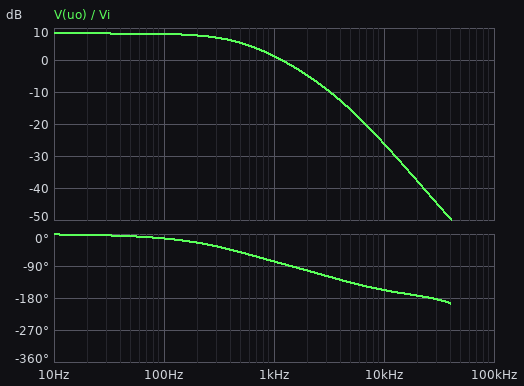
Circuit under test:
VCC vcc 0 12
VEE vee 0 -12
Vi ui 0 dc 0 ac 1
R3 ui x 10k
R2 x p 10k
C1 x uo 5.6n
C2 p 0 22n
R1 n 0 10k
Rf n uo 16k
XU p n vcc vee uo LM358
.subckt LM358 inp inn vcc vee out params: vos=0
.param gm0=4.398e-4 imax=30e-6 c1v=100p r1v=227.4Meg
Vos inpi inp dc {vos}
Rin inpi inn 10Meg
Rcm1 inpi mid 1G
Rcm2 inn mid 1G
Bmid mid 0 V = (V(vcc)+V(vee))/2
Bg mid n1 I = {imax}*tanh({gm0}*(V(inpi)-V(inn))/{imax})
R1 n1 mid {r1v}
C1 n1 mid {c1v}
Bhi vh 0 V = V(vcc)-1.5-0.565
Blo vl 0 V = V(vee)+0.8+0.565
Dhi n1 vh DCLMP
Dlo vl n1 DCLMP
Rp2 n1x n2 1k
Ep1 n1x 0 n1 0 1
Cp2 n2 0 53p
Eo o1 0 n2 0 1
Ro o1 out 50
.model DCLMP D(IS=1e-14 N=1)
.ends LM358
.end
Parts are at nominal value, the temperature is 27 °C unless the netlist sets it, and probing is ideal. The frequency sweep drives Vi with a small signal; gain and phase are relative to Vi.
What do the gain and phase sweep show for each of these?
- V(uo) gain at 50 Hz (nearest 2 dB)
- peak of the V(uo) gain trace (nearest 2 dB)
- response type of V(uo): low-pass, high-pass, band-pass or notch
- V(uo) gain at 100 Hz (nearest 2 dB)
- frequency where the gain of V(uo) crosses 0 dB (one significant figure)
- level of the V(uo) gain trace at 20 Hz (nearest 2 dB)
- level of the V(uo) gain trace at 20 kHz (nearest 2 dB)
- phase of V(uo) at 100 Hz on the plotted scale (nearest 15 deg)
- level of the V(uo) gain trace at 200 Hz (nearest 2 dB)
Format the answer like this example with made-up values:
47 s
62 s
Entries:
8 dB
8 dB
low-pass
8 dB
1 kHz
8 dB
-38 dB
-15 deg
8 dB
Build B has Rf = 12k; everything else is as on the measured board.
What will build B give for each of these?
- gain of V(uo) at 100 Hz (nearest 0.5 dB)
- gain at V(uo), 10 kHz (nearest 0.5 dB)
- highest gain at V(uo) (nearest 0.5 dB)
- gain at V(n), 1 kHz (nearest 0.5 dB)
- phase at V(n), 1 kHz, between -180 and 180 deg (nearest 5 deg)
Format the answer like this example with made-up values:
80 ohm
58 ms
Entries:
6.5 dB
-27.5 dB
7.0 dB
-7.5 dB
-80 deg
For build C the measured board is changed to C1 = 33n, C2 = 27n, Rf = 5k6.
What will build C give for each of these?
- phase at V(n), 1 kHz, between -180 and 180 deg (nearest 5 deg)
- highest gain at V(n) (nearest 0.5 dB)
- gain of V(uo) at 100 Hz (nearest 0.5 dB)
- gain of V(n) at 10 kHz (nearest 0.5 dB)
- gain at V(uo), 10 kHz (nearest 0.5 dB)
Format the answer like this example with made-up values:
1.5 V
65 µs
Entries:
-140 deg
0.5 dB
4.0 dB
-51.0 dB
-47.0 dB
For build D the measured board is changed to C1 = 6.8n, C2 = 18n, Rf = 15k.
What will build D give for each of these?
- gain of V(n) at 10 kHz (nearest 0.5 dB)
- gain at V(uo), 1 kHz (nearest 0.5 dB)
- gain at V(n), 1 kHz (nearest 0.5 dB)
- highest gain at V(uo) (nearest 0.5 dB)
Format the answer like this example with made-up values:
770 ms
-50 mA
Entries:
-34.0 dB
3.5 dB
-4.5 dB
8.0 dB
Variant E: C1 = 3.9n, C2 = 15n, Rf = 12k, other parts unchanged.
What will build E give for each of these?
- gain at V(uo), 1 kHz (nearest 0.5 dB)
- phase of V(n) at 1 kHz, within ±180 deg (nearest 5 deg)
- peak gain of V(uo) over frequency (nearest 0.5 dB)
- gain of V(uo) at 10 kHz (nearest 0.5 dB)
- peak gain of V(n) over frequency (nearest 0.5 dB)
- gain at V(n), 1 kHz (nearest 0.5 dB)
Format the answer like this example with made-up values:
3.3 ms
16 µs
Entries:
2.0 dB
-65 deg
7.0 dB
-22.0 dB
0 dB
-5.0 dB
